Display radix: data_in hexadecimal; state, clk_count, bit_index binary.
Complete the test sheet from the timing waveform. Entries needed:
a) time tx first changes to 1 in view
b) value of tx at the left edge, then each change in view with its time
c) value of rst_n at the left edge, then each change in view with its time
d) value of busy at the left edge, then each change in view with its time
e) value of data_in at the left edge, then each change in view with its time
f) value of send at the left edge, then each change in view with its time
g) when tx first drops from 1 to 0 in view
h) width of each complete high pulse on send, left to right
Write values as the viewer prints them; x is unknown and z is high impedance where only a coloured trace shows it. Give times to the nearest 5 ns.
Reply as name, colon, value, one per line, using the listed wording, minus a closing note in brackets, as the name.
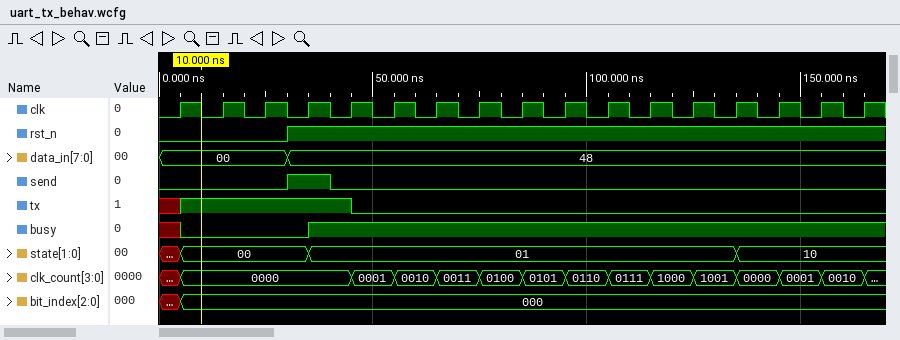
time tx first changes to 1 in view: 5 ns
value of tx at the left edge, then each change in view with its time: x, 1 at 5 ns, 0 at 45 ns
value of rst_n at the left edge, then each change in view with its time: 0, 1 at 30 ns
value of busy at the left edge, then each change in view with its time: x, 0 at 5 ns, 1 at 35 ns
value of data_in at the left edge, then each change in view with its time: 00, 48 at 30 ns
value of send at the left edge, then each change in view with its time: 0, 1 at 30 ns, 0 at 40 ns
when tx first drops from 1 to 0 in view: 45 ns
width of each complete high pulse on send, left to right: 10 ns
